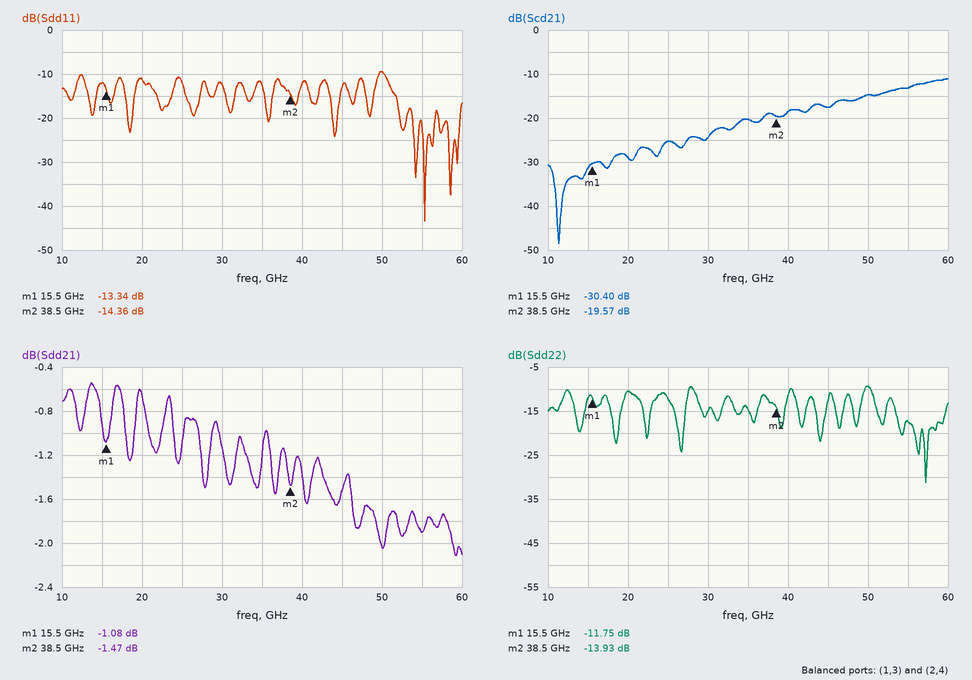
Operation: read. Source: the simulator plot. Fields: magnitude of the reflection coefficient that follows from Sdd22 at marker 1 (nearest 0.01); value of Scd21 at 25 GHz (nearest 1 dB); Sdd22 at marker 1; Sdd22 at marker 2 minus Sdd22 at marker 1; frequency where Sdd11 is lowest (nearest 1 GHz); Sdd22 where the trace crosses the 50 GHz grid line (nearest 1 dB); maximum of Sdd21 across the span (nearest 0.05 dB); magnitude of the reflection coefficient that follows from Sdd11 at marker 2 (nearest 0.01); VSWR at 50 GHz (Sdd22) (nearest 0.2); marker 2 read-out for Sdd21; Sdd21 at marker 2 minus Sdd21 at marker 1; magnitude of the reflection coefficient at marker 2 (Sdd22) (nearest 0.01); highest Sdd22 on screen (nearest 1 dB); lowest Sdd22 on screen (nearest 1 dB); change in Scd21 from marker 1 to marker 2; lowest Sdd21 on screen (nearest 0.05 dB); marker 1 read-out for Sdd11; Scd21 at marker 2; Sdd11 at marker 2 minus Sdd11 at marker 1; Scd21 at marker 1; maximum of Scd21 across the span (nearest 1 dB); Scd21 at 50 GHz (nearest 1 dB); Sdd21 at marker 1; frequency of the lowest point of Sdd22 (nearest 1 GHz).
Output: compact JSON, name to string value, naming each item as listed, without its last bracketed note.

{"magnitude of the reflection coefficient that follows from Sdd22 at marker 1": "0.26", "value of Scd21 at 25 GHz": "-25 dB", "Sdd22 at marker 1": "-11.75 dB", "Sdd22 at marker 2 minus Sdd22 at marker 1": "-2.18 dB", "frequency where Sdd11 is lowest": "55 GHz", "Sdd22 where the trace crosses the 50 GHz grid line": "-9 dB", "maximum of Sdd21 across the span": "-0.55 dB", "magnitude of the reflection coefficient that follows from Sdd11 at marker 2": "0.19", "VSWR at 50 GHz (Sdd22)": "2.0", "marker 2 read-out for Sdd21": "-1.47 dB", "Sdd21 at marker 2 minus Sdd21 at marker 1": "-0.39 dB", "magnitude of the reflection coefficient at marker 2 (Sdd22)": "0.20", "highest Sdd22 on screen": "-9 dB", "lowest Sdd22 on screen": "-31 dB", "change in Scd21 from marker 1 to marker 2": "10.83 dB", "lowest Sdd21 on screen": "-2.10 dB", "marker 1 read-out for Sdd11": "-13.34 dB", "Scd21 at marker 2": "-19.57 dB", "Sdd11 at marker 2 minus Sdd11 at marker 1": "-1.02 dB", "Scd21 at marker 1": "-30.40 dB", "maximum of Scd21 across the span": "-11 dB", "Scd21 at 50 GHz": "-15 dB", "Sdd21 at marker 1": "-1.08 dB", "frequency of the lowest point of Sdd22": "57 GHz"}
